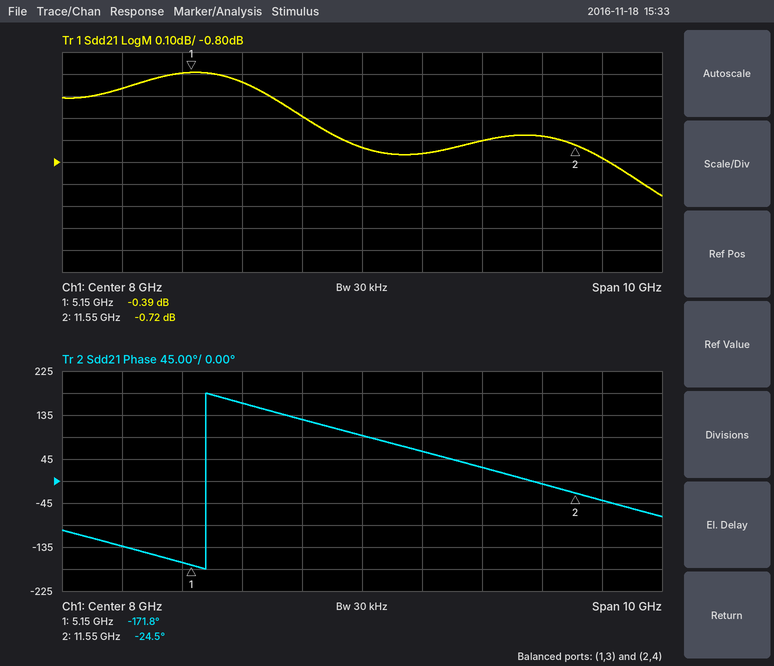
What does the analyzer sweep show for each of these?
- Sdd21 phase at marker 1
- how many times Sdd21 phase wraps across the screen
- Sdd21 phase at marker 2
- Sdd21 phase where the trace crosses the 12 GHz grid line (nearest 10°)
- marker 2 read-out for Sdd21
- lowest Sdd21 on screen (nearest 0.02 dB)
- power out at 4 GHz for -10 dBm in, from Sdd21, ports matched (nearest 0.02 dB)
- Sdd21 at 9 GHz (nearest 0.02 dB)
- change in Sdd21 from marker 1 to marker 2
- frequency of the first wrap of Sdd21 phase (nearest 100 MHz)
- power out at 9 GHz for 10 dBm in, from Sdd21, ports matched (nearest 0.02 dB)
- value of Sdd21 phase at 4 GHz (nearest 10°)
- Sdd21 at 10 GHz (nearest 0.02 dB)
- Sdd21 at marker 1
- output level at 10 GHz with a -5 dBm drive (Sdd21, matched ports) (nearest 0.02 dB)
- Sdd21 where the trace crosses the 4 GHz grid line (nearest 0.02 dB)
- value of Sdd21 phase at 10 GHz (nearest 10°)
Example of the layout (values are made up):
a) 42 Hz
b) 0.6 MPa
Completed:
a) -171.8°
b) 1
c) -24.5°
d) -40°
e) -0.72 dB
f) -0.96 dB
g) -10.46 dBm
h) -0.76 dB
i) -0.33 dB
j) 5.4 GHz
k) 9.24 dBm
l) -130°
m) -0.70 dB
n) -0.39 dB
o) -5.70 dBm
p) -0.46 dB
q) 30°
